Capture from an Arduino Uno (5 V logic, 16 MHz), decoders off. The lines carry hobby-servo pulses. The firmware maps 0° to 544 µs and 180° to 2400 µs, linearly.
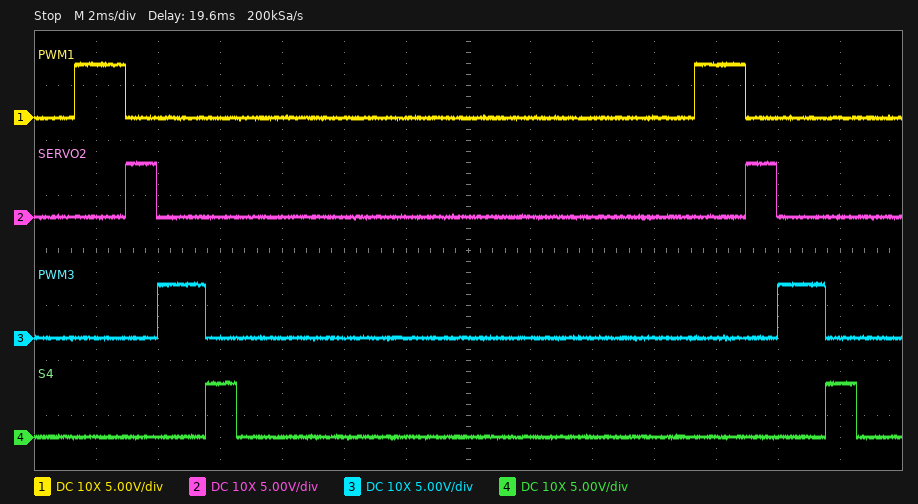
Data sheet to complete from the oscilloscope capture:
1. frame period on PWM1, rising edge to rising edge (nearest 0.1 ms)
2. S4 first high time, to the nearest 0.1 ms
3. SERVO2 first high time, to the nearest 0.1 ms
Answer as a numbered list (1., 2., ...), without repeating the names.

1. 20.0 ms
2. 1.0 ms
3. 1.0 ms
